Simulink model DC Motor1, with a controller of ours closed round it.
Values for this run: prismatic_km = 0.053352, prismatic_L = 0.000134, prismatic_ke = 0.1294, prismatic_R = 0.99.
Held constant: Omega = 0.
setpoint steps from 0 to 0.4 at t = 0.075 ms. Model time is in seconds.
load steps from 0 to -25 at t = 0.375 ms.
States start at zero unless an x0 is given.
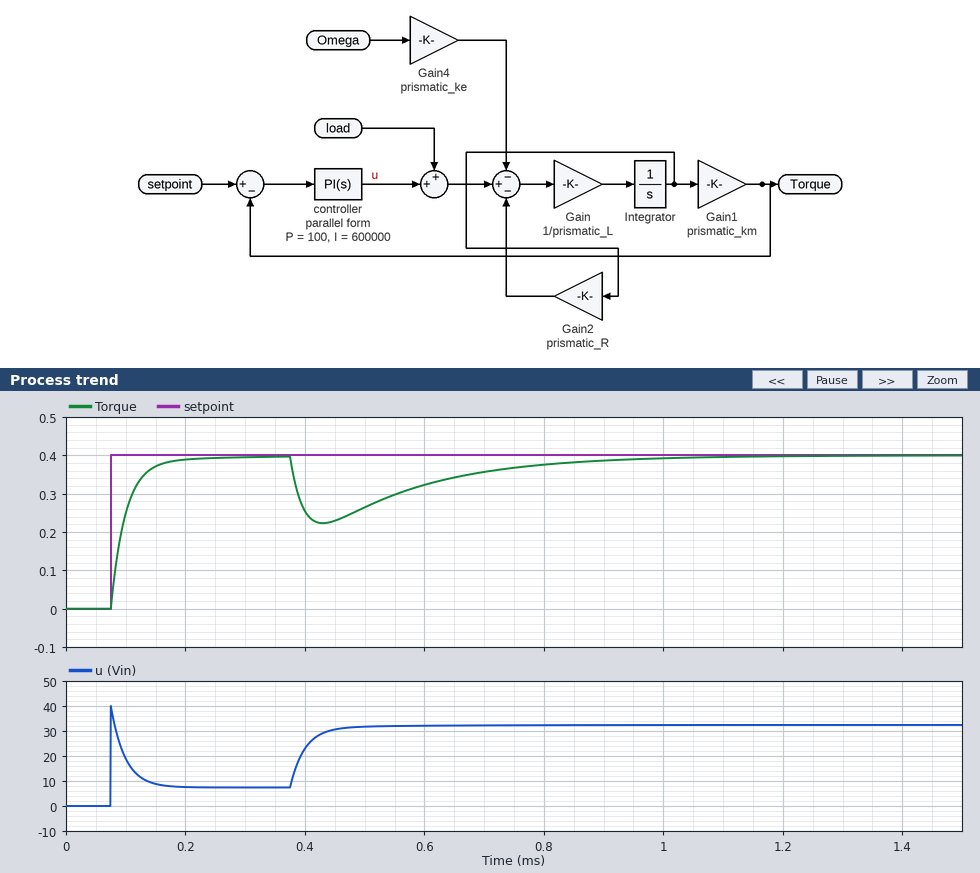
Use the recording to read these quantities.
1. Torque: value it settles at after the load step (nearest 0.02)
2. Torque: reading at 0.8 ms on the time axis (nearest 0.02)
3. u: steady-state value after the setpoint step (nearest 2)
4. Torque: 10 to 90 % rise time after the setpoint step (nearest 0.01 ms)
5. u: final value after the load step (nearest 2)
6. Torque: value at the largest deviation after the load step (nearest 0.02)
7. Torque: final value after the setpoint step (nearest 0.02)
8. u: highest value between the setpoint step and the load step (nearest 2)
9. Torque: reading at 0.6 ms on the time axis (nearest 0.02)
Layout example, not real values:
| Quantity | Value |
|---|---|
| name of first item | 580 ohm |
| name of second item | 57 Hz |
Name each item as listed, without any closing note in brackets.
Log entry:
| Quantity | Value |
|---|---|
| Torque: value it settles at after the load step | 0.40 |
| Torque: reading at 0.8 ms on the time axis | 0.38 |
| u: steady-state value after the setpoint step | 8 |
| Torque: 10 to 90 % rise time after the setpoint step | 0.06 ms |
| u: final value after the load step | 32 |
| Torque: value at the largest deviation after the load step | 0.22 |
| Torque: final value after the setpoint step | 0.40 |
| u: highest value between the setpoint step and the load step | 40 |
| Torque: reading at 0.6 ms on the time axis | 0.32 |
